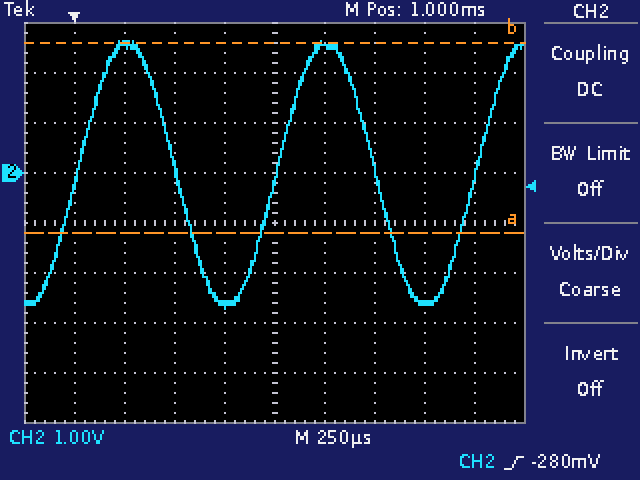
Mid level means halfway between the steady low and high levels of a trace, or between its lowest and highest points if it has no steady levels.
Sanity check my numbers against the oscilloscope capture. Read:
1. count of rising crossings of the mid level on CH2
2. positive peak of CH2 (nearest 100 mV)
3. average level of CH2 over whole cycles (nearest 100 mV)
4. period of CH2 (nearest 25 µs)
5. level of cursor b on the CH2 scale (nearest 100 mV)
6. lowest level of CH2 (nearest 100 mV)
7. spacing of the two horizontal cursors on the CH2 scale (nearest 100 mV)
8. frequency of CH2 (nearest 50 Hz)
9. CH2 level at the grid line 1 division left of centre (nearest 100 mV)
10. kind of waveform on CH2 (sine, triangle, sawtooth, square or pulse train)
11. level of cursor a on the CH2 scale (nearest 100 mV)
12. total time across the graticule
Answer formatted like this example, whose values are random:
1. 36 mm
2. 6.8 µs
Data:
1. 3
2. 2.6 V
3. 0.0 V
4. 1.000 ms
5. 2.6 V
6. -2.7 V
7. 3.8 V
8. 1.00 kHz
9. -2.6 V
10. sine
11. -1.2 V
12. 2.5 ms
